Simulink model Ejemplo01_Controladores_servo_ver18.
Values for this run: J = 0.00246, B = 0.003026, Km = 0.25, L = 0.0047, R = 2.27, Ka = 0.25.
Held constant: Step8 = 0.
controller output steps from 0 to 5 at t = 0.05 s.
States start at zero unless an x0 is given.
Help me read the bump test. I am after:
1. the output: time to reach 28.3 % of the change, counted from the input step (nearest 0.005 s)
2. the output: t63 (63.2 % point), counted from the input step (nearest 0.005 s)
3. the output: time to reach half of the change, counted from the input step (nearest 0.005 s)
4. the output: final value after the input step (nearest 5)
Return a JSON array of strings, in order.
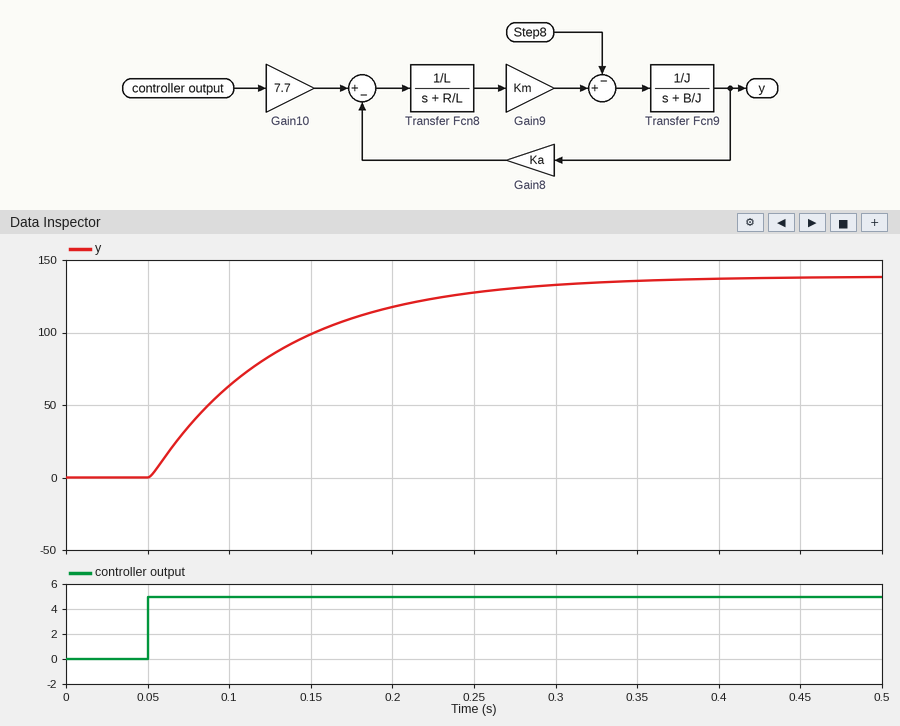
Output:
["0.030 s", "0.080 s", "0.055 s", "140"]
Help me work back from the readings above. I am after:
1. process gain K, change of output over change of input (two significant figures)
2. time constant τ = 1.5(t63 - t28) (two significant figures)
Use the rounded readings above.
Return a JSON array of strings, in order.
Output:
["28", "0.075 s"]
